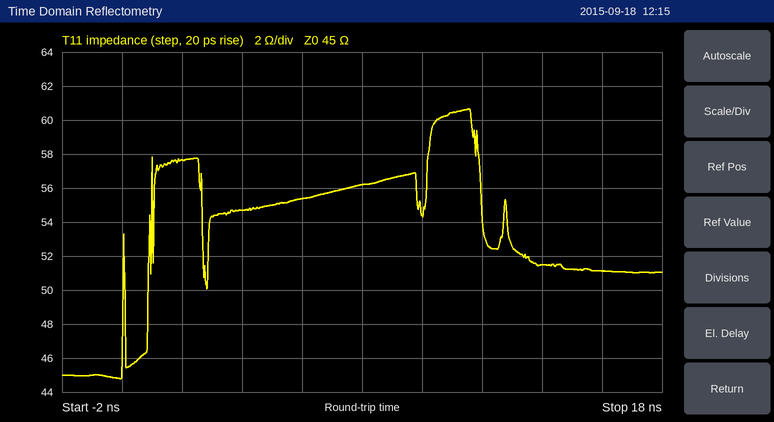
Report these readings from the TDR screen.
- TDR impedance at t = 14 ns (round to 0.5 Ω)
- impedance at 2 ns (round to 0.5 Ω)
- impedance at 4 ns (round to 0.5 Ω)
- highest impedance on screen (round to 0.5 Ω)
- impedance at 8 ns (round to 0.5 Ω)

51.5 Ω
57.5 Ω
54.5 Ω
60.5 Ω
56.0 Ω
